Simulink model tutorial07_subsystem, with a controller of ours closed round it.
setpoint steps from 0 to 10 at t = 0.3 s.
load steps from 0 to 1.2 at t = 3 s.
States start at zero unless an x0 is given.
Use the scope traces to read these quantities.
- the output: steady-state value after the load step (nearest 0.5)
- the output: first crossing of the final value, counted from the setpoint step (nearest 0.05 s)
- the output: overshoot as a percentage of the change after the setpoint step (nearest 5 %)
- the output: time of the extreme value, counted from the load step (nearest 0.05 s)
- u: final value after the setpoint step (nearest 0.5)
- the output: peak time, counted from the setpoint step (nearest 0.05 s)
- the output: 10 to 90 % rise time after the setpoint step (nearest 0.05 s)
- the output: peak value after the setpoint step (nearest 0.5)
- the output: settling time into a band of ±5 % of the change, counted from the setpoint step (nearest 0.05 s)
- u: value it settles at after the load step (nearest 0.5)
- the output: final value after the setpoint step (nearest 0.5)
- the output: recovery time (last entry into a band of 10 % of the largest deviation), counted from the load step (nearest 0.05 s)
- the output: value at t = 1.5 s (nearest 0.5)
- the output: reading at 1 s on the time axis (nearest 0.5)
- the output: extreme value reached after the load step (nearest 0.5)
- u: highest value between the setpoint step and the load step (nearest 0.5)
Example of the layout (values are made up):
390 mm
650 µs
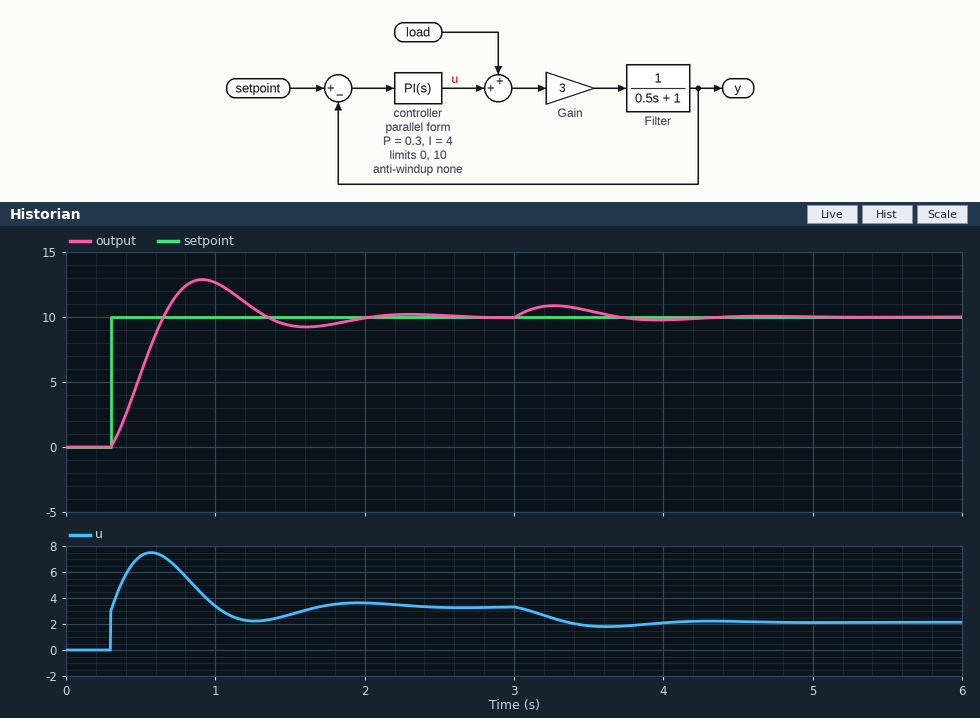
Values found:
10.0
0.35 s
30 %
0.25 s
3.5
0.60 s
0.25 s
13.0
1.50 s
2.0
10.0
1.25 s
9.5
12.5
11.0
7.5
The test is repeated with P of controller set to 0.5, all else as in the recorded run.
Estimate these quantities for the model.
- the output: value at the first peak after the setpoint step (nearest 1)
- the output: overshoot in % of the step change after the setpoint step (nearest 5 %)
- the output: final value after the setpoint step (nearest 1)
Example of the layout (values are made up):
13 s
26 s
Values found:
12
20 %
10
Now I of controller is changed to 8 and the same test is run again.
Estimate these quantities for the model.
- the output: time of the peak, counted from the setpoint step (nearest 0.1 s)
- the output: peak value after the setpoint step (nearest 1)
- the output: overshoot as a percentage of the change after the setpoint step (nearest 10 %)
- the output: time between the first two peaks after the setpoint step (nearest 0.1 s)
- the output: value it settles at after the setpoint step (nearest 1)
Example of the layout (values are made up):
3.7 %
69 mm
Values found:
0.4 s
14
40 %
0.9 s
10
